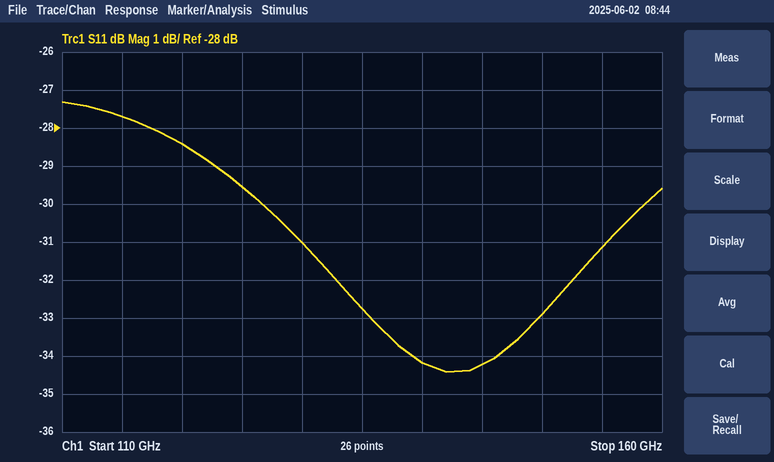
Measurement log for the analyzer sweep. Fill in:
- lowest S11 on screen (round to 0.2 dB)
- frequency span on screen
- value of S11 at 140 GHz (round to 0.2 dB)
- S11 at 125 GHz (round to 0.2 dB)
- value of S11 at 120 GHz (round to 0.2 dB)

-34.4 dB
50 GHz
-34.2 dB
-29.6 dB
-28.4 dB
